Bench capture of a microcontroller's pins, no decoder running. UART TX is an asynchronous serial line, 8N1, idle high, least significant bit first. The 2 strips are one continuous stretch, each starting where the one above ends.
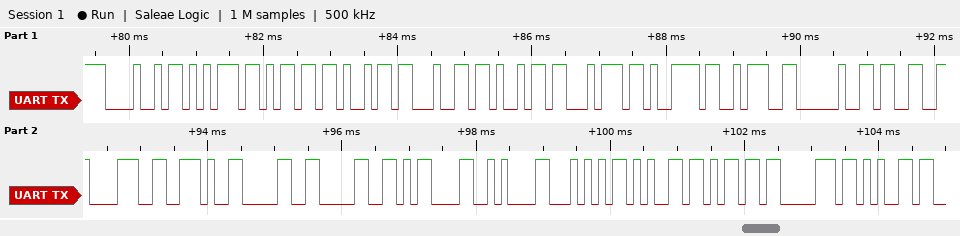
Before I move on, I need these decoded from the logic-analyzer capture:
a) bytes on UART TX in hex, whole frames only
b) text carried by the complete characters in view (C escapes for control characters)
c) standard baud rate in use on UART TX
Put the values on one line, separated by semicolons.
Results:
48 75 6D 69 64 69 74 79 3A 20 33 38 2E 30 30 0D 0A 54 65 6D 70 65; "Humidity: 38.00\r\nTempe"; 9600 baud
